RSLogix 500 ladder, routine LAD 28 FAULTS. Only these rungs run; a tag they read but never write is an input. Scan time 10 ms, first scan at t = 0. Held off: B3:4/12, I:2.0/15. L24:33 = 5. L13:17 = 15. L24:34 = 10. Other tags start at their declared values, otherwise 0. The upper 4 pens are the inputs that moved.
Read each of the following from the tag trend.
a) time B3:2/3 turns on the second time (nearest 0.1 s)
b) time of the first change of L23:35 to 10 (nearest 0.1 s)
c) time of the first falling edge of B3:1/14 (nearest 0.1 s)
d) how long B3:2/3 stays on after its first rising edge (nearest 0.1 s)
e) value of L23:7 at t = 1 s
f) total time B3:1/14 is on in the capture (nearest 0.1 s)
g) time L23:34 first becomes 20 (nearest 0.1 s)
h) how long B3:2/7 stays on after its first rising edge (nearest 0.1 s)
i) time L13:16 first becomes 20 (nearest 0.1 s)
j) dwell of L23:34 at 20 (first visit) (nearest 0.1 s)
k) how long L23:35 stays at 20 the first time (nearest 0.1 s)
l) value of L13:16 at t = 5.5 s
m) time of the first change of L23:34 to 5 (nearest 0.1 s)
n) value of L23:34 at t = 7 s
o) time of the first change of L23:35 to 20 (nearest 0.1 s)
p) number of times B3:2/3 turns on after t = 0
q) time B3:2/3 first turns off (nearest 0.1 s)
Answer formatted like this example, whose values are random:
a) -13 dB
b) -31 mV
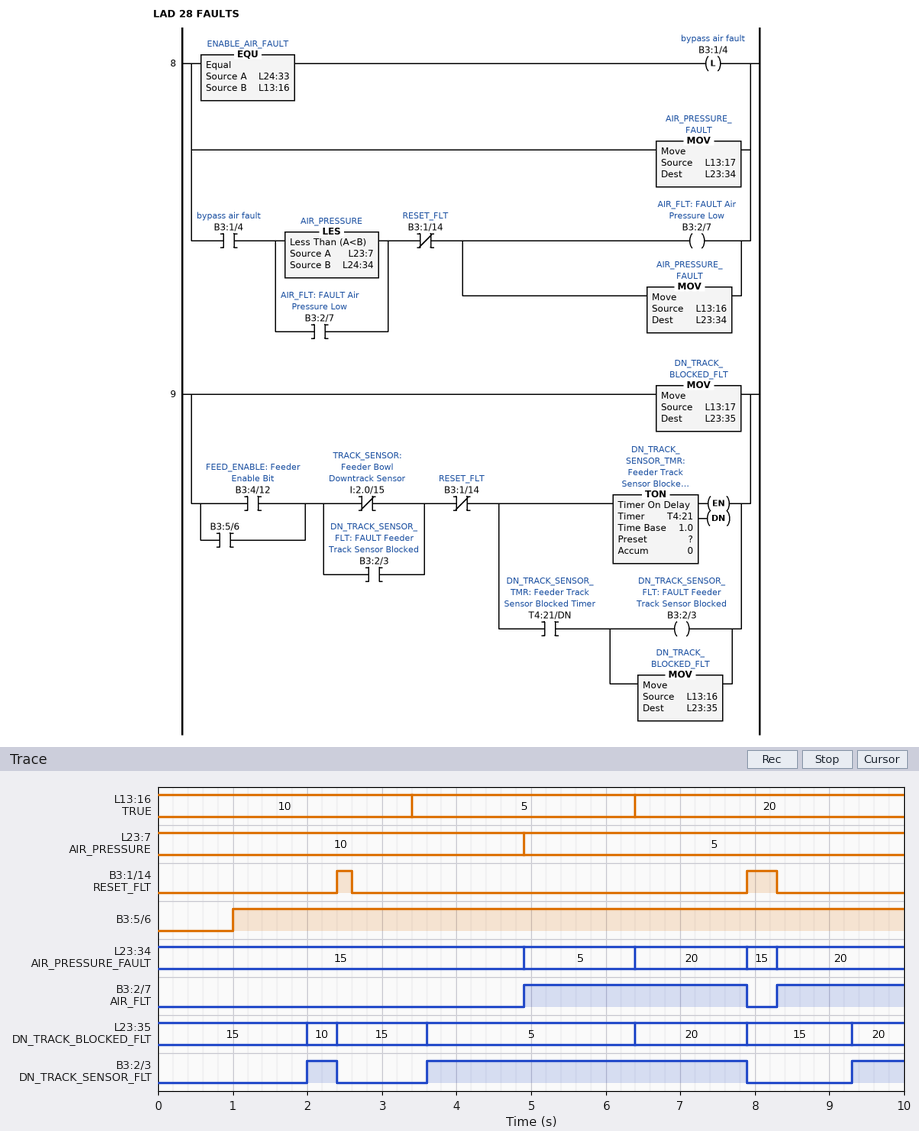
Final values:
a) 3.6 s
b) 2.0 s
c) 2.6 s
d) 0.4 s
e) 10
f) 0.6 s
g) 6.4 s
h) 3.0 s
i) 6.4 s
j) 1.5 s
k) 1.5 s
l) 5
m) 4.9 s
n) 20
o) 6.4 s
p) 3
q) 2.4 s
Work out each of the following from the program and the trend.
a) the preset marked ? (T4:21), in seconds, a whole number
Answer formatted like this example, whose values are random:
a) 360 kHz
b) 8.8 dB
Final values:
a) 1 s
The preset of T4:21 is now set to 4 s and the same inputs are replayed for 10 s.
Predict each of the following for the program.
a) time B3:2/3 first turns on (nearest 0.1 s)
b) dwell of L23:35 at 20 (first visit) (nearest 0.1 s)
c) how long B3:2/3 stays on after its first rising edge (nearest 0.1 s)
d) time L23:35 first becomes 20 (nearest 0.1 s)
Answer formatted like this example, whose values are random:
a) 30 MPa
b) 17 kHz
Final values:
a) 6.6 s
b) 1.3 s
c) 1.3 s
d) 6.6 s
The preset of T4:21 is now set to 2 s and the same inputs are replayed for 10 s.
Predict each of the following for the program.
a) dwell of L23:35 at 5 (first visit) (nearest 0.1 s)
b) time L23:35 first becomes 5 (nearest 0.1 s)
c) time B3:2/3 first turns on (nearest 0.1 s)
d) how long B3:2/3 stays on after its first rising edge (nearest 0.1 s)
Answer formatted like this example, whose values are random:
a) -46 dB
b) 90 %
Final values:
a) 1.8 s
b) 4.6 s
c) 4.6 s
d) 3.3 s
